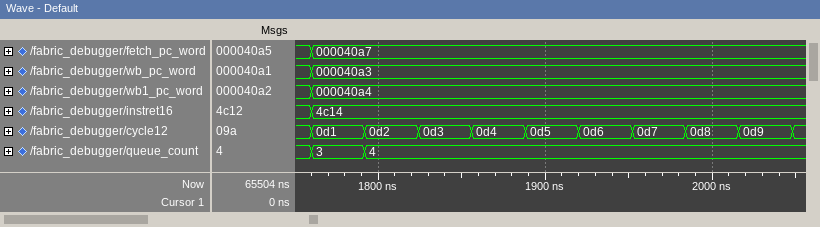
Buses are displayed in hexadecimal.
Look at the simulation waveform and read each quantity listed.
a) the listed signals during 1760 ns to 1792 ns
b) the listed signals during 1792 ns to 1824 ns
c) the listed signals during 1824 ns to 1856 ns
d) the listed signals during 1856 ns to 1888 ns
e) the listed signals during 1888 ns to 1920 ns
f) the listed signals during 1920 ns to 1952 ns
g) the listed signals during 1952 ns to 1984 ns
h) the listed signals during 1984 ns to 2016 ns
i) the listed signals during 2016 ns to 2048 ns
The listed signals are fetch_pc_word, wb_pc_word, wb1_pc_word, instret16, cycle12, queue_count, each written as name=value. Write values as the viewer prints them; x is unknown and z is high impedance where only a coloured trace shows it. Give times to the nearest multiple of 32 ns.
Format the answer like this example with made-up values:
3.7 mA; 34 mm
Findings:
fetch_pc_word=000040a7, wb_pc_word=000040a3, wb1_pc_word=000040a4, instret16=4c14, cycle12=0d1, queue_count=3; fetch_pc_word=000040a7, wb_pc_word=000040a3, wb1_pc_word=000040a4, instret16=4c14, cycle12=0d2, queue_count=4; fetch_pc_word=000040a7, wb_pc_word=000040a3, wb1_pc_word=000040a4, instret16=4c14, cycle12=0d3, queue_count=4; fetch_pc_word=000040a7, wb_pc_word=000040a3, wb1_pc_word=000040a4, instret16=4c14, cycle12=0d4, queue_count=4; fetch_pc_word=000040a7, wb_pc_word=000040a3, wb1_pc_word=000040a4, instret16=4c14, cycle12=0d5, queue_count=4; fetch_pc_word=000040a7, wb_pc_word=000040a3, wb1_pc_word=000040a4, instret16=4c14, cycle12=0d6, queue_count=4; fetch_pc_word=000040a7, wb_pc_word=000040a3, wb1_pc_word=000040a4, instret16=4c14, cycle12=0d7, queue_count=4; fetch_pc_word=000040a7, wb_pc_word=000040a3, wb1_pc_word=000040a4, instret16=4c14, cycle12=0d8, queue_count=4; fetch_pc_word=000040a7, wb_pc_word=000040a3, wb1_pc_word=000040a4, instret16=4c14, cycle12=0d9, queue_count=4
